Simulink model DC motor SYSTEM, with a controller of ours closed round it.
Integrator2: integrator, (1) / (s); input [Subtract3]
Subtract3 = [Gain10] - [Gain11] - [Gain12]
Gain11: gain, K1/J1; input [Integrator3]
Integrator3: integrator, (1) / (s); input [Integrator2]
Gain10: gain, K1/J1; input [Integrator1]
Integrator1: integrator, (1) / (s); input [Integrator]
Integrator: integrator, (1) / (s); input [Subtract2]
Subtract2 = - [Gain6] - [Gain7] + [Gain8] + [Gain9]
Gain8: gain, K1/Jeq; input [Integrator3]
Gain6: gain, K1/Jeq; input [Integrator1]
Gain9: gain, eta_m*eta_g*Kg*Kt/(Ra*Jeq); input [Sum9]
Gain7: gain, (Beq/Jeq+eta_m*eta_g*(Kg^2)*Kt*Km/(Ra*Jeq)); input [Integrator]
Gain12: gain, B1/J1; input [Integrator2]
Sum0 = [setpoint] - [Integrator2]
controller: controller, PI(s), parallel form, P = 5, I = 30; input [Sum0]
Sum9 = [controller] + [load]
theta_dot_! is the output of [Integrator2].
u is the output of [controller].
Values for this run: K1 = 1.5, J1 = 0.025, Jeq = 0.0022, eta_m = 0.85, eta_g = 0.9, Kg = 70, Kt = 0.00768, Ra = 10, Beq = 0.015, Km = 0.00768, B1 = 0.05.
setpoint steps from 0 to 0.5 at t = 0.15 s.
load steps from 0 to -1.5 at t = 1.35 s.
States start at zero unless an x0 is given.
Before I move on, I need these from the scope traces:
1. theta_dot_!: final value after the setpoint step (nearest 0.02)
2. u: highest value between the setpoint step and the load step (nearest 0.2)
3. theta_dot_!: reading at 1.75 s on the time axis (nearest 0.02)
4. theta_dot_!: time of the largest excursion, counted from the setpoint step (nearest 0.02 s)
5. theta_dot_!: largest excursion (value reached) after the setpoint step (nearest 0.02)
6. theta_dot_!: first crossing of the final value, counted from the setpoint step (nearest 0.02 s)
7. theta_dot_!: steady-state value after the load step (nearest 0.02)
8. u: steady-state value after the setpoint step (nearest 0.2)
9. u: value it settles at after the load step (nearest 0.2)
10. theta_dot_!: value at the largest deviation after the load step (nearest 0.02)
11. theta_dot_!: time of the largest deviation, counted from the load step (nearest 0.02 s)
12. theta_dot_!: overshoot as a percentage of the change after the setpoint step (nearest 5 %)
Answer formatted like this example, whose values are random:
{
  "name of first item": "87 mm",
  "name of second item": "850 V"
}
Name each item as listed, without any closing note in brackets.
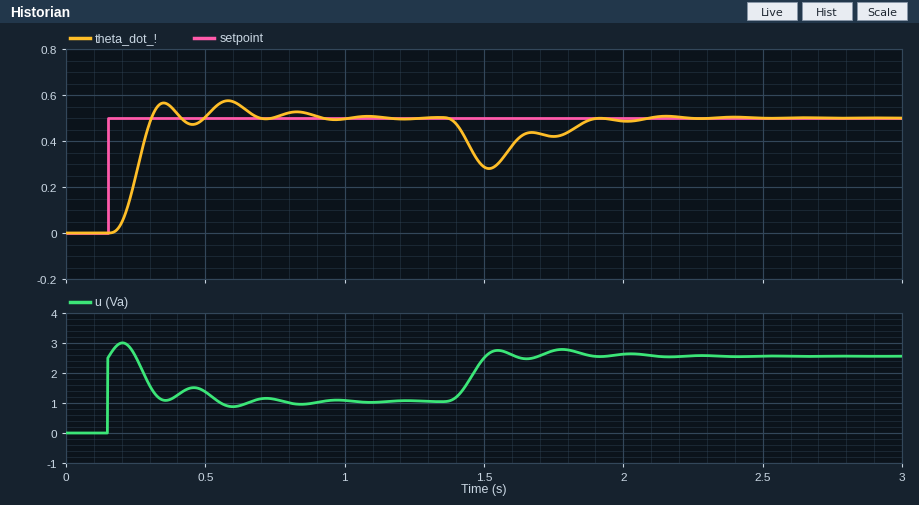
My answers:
{
  "theta_dot_!: final value after the setpoint step": "0.50",
  "u: highest value between the setpoint step and the load step": "3.0",
  "theta_dot_!: reading at 1.75 s on the time axis": "0.42",
  "theta_dot_!: time of the largest excursion, counted from the setpoint step": "0.44 s",
  "theta_dot_!: largest excursion (value reached) after the setpoint step": "0.58",
  "theta_dot_!: first crossing of the final value, counted from the setpoint step": "0.16 s",
  "theta_dot_!: steady-state value after the load step": "0.50",
  "u: steady-state value after the setpoint step": "1.0",
  "u: value it settles at after the load step": "2.6",
  "theta_dot_!: value at the largest deviation after the load step": "0.28",
  "theta_dot_!: time of the largest deviation, counted from the load step": "0.16 s",
  "theta_dot_!: overshoot as a percentage of the change after the setpoint step": "15 %"
}
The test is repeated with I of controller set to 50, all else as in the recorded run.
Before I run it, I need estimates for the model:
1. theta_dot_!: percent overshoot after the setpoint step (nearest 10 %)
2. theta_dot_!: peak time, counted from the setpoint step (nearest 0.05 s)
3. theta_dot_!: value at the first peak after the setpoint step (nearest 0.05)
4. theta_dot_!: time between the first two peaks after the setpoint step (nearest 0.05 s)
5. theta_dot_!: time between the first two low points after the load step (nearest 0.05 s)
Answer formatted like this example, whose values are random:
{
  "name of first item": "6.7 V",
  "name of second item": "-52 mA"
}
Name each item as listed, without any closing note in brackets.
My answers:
{
  "theta_dot_!: percent overshoot after the setpoint step": "40 %",
  "theta_dot_!: peak time, counted from the setpoint step": "0.20 s",
  "theta_dot_!: value at the first peak after the setpoint step": "0.70",
  "theta_dot_!: time between the first two peaks after the setpoint step": "0.25 s",
  "theta_dot_!: time between the first two low points after the load step": "0.25 s"
}
